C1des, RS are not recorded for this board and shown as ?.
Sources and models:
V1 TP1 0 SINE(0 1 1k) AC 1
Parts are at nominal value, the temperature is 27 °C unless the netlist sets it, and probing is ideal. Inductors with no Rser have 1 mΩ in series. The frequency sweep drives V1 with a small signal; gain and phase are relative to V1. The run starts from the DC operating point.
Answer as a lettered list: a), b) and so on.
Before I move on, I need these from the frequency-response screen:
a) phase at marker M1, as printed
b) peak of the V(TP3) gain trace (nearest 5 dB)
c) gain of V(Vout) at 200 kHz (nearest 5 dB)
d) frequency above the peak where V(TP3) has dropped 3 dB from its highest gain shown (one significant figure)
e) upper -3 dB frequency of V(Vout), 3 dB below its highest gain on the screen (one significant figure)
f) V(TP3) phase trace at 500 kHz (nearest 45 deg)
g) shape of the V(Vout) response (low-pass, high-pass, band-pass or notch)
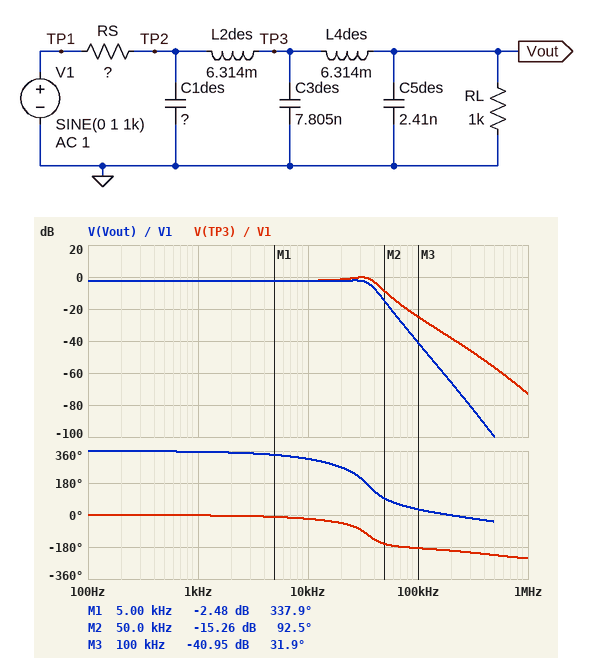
a) 337.9 deg
b) 0 dB
c) -65 dB
d) 40 kHz
e) 40 kHz
f) -225 deg
g) low-pass
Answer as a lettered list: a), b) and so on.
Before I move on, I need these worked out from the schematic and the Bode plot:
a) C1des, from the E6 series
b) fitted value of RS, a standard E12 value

a) 1 nF
b) 330 Ω
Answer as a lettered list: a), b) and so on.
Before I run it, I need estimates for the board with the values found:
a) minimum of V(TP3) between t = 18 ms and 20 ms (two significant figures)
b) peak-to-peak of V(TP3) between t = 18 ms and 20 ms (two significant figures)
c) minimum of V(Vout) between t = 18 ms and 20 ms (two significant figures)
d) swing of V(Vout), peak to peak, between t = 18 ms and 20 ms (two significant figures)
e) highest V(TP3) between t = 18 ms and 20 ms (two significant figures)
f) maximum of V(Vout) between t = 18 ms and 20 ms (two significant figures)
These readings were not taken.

a) -750 mV
b) 1.5 V
c) -750 mV
d) 1.5 V
e) 750 mV
f) 750 mV
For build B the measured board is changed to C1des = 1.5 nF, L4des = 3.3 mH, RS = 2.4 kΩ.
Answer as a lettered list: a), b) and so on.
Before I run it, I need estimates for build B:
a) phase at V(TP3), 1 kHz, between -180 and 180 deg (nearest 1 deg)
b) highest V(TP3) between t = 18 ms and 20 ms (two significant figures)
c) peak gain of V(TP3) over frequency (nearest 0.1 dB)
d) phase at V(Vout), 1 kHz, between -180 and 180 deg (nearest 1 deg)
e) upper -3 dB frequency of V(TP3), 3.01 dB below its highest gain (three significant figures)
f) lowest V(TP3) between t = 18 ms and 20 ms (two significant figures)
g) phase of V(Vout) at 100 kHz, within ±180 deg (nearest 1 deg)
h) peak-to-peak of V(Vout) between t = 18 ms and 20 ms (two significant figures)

a) -3 deg
b) 290 mV
c) -10.6 dB
d) -4 deg
e) 61.1 kHz
f) -290 mV
g) -13 deg
h) 590 mV
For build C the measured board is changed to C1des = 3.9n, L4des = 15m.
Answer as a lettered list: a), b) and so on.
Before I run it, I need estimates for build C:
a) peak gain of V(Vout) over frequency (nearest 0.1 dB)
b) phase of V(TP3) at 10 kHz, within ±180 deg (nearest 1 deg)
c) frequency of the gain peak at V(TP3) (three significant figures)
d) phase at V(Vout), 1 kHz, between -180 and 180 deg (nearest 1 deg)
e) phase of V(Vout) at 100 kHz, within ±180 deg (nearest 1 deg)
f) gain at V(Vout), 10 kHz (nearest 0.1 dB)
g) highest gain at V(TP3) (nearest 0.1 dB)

a) -1.6 dB
b) -15 deg
c) 27.6 kHz
d) -7 deg
e) 0 deg
f) -3.9 dB
g) 6.6 dB
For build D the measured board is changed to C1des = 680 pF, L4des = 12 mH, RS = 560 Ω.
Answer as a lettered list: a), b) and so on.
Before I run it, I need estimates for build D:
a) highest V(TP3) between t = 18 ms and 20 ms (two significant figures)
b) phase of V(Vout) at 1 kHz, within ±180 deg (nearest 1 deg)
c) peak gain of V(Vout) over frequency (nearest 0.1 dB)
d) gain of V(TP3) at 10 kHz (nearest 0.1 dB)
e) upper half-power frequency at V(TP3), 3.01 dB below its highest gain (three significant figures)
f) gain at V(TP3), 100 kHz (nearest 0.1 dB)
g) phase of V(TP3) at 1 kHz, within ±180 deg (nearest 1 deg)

a) 640 mV
b) -6 deg
c) -3.8 dB
d) -3.1 dB
e) 34.2 kHz
f) -25.1 dB
g) -1 deg
